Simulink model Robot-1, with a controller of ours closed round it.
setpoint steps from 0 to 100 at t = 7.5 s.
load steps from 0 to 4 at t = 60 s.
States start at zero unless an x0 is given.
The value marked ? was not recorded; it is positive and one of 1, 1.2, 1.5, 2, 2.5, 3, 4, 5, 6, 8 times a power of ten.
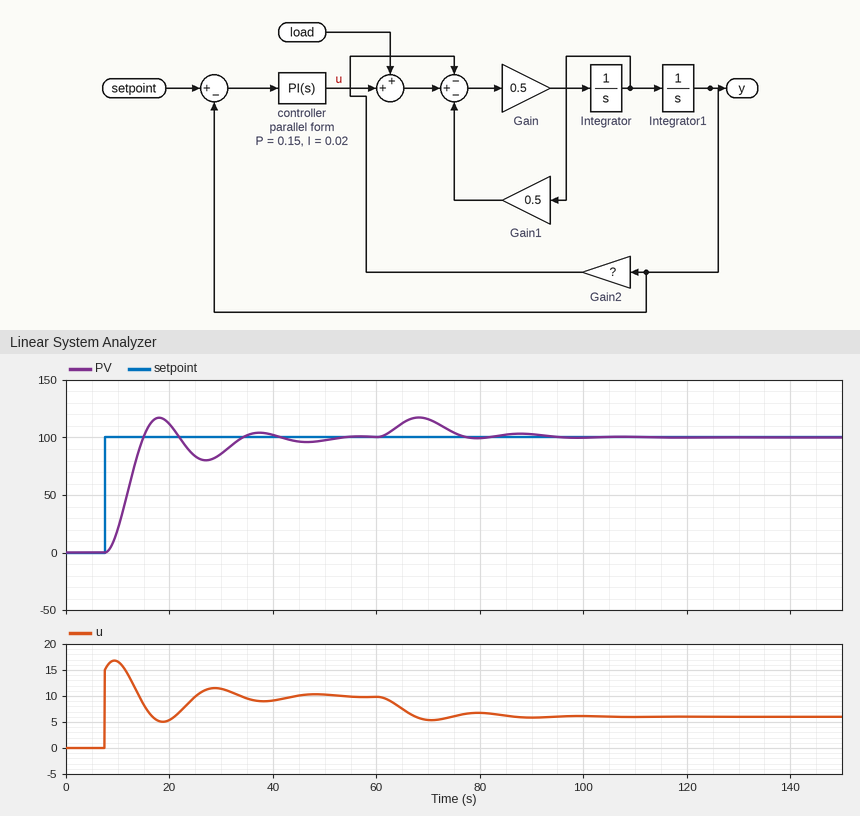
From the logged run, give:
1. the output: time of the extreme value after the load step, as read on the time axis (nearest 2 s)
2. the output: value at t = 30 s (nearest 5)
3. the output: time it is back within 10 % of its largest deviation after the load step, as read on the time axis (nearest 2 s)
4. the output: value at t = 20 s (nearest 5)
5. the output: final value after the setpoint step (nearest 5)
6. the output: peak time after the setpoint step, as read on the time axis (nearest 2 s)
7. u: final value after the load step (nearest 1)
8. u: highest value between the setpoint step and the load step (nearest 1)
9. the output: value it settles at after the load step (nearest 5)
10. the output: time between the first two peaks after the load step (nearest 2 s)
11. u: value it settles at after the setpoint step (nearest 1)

68 s
85
92 s
110
100
18 s
6
17
100
20 s
10
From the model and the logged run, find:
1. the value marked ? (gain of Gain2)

0.1
